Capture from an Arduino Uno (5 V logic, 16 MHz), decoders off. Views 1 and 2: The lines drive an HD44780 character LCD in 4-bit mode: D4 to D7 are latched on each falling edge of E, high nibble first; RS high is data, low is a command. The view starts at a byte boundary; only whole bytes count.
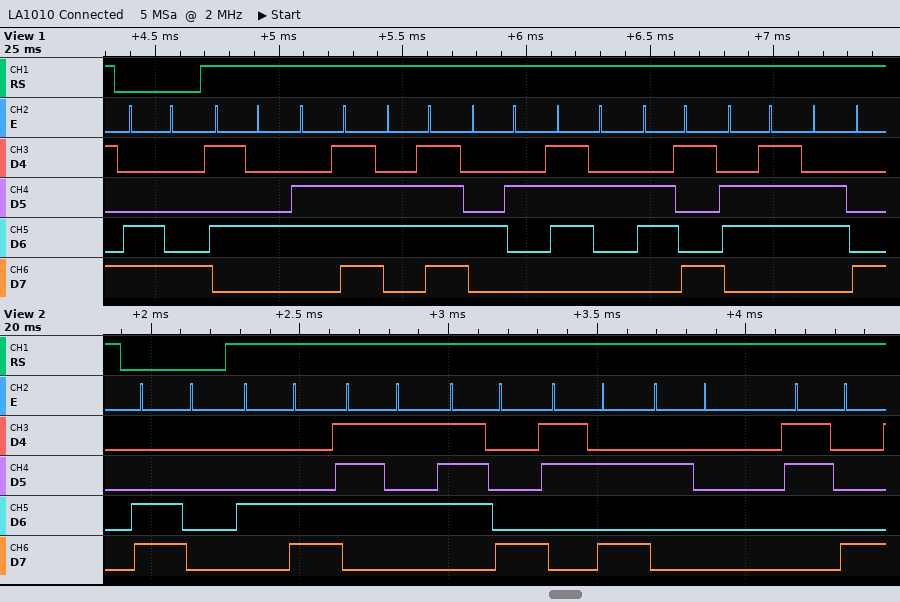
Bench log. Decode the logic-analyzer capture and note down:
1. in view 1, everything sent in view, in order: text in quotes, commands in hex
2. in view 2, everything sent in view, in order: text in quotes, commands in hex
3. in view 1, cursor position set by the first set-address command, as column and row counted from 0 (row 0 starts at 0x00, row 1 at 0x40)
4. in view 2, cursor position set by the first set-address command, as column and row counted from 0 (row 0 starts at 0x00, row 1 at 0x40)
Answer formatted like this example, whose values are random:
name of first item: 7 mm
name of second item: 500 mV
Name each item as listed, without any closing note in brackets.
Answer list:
in view 1, everything sent in view, in order: text in quotes, commands in hex: 0xC8 "TooBrigh"
in view 2, everything sent in view, in order: text in quotes, commands in hex: 0xC0 "Lux: 8"
in view 1, cursor position set by the first set-address command, as column and row counted from 0: column 8, row 1
in view 2, cursor position set by the first set-address command, as column and row counted from 0: column 0, row 1
